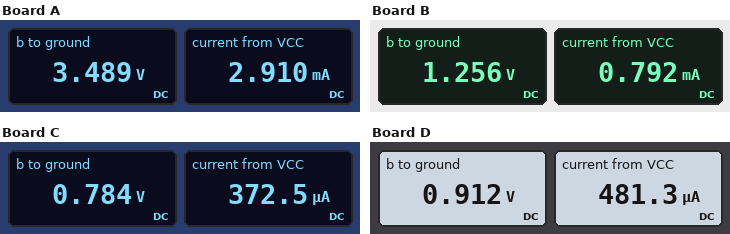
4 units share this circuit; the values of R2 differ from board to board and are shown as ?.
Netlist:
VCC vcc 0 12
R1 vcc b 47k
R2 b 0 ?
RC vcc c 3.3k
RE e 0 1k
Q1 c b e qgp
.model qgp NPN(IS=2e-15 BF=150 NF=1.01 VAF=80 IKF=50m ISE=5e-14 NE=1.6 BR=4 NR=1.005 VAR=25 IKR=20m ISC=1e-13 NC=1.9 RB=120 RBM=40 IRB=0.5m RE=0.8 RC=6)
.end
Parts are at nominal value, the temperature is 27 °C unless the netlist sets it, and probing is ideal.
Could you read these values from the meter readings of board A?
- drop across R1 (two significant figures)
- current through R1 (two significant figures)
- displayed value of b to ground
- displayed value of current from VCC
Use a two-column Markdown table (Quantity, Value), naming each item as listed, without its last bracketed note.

| Quantity | Value |
|---|---|
| drop across R1 | 8.5 V |
| current through R1 | 180 µA |
| displayed value of b to ground | 3.489 V |
| displayed value of current from VCC | 2.910 mA |
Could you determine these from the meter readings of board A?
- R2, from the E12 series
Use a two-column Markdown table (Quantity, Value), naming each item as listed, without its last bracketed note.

| Quantity | Value |
|---|---|
| R2, from the E12 series | 22 kΩ |
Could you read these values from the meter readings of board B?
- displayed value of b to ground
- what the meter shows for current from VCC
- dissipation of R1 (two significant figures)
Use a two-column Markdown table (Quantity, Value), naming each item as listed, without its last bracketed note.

| Quantity | Value |
|---|---|
| displayed value of b to ground | 1.256 V |
| what the meter shows for current from VCC | 0.792 mA |
| dissipation of R1 | 2.5 mW |
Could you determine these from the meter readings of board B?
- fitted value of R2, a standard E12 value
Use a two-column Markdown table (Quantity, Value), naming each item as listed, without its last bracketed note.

| Quantity | Value |
|---|---|
| fitted value of R2, a standard E12 value | 5.6 kΩ |
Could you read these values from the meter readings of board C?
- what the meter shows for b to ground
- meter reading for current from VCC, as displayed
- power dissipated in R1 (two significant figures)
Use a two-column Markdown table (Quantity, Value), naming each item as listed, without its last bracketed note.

| Quantity | Value |
|---|---|
| what the meter shows for b to ground | 0.784 V |
| meter reading for current from VCC, as displayed | 372.5 µA |
| power dissipated in R1 | 2.7 mW |
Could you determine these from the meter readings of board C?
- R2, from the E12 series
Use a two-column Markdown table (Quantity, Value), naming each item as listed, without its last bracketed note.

| Quantity | Value |
|---|---|
| R2, from the E12 series | 3.3 kΩ |
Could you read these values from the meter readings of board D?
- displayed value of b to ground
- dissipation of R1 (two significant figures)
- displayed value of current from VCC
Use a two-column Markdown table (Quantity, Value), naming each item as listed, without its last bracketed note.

| Quantity | Value |
|---|---|
| displayed value of b to ground | 0.912 V |
| dissipation of R1 | 2.6 mW |
| displayed value of current from VCC | 481.3 µA |
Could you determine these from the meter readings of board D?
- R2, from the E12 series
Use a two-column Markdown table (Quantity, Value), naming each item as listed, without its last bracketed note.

| Quantity | Value |
|---|---|
| R2, from the E12 series | 3.9 kΩ |
